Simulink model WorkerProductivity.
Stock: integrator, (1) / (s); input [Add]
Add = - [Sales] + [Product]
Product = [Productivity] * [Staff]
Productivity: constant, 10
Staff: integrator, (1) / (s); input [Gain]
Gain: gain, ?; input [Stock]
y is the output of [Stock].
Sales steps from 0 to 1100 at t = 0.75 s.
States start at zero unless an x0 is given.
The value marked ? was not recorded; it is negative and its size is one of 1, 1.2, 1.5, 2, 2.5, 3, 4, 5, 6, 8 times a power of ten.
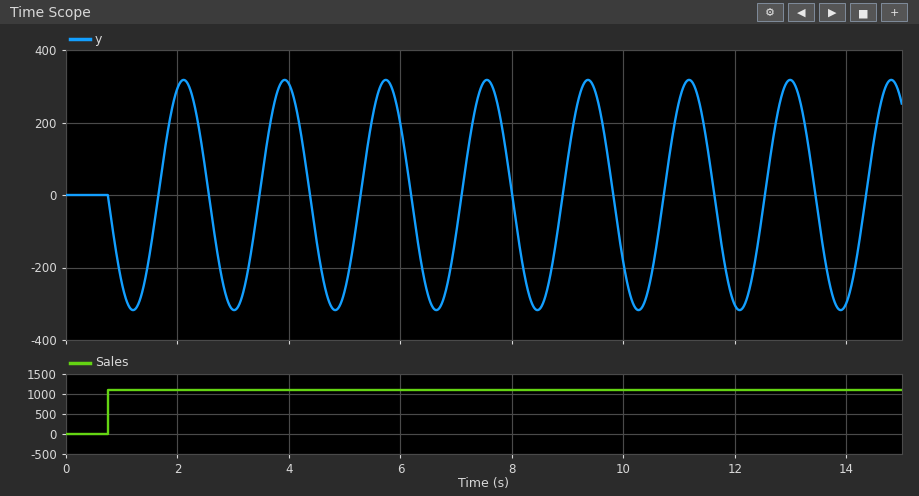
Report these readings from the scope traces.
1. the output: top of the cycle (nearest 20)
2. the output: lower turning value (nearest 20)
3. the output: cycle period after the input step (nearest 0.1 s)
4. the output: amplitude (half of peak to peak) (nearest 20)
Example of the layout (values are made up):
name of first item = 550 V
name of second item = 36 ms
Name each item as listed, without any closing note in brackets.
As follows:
the output: top of the cycle = 320
the output: lower turning value = -320
the output: cycle period after the input step = 1.8 s
the output: amplitude (half of peak to peak) = 320
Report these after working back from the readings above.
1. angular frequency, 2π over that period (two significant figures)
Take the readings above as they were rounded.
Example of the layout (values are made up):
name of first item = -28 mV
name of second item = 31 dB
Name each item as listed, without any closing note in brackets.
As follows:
angular frequency, 2π over that period = 3.5 rad/s
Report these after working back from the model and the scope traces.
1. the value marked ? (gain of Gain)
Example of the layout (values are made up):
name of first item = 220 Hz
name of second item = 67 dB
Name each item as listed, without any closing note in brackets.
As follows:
the value marked ? = -1.2
